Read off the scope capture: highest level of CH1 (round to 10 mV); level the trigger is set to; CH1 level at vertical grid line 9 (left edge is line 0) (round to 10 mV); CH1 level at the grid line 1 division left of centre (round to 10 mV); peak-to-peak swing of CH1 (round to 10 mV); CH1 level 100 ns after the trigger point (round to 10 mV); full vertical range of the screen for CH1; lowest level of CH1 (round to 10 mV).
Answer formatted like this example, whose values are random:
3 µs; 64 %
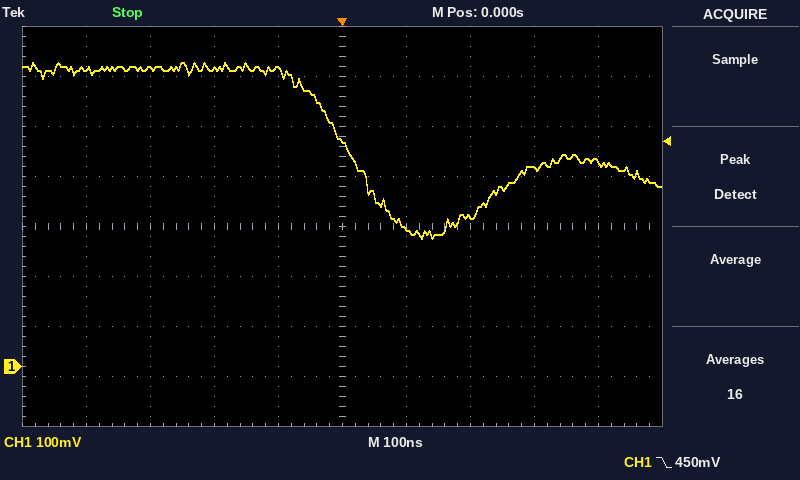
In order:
610 mV; 450 mV; 410 mV; 600 mV; 350 mV; 280 mV; 800 mV; 260 mV
